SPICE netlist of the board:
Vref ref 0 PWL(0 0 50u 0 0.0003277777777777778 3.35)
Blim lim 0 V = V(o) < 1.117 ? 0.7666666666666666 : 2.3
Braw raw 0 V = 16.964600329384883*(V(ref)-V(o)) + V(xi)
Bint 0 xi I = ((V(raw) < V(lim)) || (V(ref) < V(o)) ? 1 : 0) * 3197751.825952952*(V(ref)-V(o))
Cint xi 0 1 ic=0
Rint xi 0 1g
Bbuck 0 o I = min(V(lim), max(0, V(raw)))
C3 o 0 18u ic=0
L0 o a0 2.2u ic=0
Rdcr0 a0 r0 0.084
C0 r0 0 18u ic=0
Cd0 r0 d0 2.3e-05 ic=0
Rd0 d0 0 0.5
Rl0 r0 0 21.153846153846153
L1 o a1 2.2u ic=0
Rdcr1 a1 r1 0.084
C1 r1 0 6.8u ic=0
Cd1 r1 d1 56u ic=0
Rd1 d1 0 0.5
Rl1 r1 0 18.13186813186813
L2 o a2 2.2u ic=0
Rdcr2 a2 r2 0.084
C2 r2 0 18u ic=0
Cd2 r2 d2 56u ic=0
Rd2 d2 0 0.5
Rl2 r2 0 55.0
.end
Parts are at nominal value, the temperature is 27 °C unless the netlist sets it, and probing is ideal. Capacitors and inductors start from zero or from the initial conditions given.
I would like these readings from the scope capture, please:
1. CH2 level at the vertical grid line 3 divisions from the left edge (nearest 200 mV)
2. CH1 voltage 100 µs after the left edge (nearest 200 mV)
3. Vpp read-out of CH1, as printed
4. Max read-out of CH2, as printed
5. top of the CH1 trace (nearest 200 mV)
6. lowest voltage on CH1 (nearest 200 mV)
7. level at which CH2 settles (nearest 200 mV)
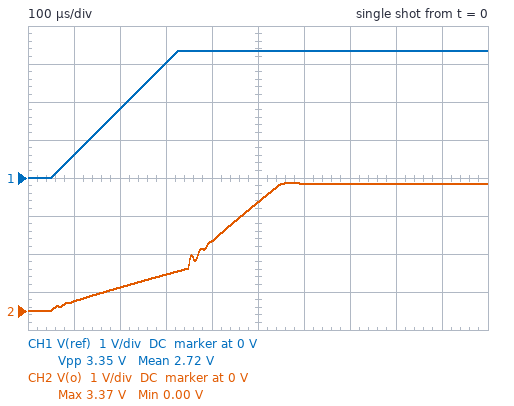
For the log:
1.0 V
600 mV
3.35 V
3.37 V
3.4 V
0 V
3.4 V
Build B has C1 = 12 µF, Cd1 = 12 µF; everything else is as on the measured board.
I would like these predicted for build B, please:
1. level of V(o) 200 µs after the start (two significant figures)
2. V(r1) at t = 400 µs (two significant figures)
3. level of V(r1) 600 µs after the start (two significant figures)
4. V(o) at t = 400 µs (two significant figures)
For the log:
740 mV
2.6 V
3.3 V
2.7 V
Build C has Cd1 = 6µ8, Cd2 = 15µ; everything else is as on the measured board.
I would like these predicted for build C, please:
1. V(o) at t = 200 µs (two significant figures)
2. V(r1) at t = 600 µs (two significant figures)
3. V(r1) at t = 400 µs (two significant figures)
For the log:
1.0 V
3.3 V
3.3 V
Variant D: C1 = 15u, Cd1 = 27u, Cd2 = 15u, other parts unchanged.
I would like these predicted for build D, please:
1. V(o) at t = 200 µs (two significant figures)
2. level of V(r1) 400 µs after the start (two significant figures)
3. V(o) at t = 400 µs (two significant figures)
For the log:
820 mV
3.2 V
3.3 V
